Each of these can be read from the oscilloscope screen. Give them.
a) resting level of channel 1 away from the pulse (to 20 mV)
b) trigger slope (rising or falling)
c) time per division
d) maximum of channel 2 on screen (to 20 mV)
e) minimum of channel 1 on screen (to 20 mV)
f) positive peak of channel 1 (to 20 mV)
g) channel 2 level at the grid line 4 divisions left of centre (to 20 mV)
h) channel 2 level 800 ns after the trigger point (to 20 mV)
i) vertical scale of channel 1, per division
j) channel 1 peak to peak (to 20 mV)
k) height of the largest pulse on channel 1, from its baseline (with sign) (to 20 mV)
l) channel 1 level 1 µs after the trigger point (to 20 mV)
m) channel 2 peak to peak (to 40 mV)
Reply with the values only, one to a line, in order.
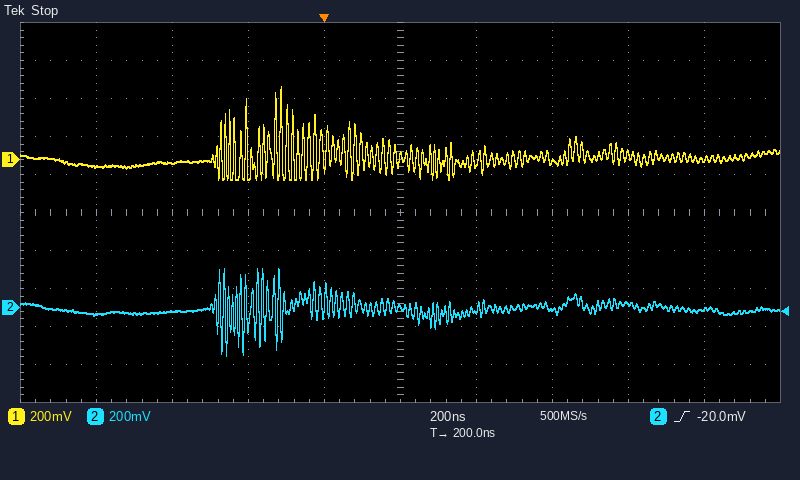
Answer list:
0 mV
rising
200 ns
200 mV
-100 mV
380 mV
-40 mV
20 mV
200 mV
480 mV
+380 mV
0 mV
440 mV
